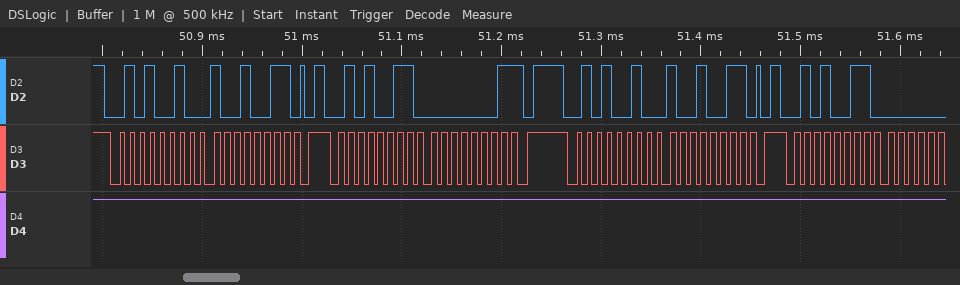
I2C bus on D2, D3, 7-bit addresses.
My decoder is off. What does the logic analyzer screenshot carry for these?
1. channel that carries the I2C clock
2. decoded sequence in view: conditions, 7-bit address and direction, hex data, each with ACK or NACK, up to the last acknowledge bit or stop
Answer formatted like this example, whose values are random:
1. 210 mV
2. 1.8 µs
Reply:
1. D3
2. start, address 29 write ACK, 93 ACK, stop, start, address 29 read ACK, 01 NACK, stop, start, address 29 write ACK, 93 ACK, stop, start, address 29 read ACK
